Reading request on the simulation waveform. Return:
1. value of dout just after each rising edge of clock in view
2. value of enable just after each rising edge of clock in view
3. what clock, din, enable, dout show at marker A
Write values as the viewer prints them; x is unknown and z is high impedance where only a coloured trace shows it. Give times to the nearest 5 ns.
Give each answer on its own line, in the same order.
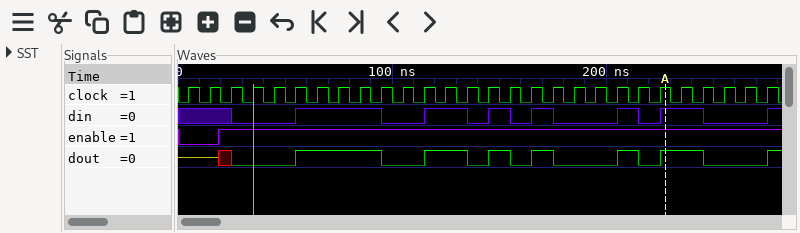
z z 0 0 0 1 1 1 1 0 0 1 1 0 1 0 1 0 0 0 1 0 1 1 0 0 0 1
0 0 1 1 1 1 1 1 1 1 1 1 1 1 1 1 1 1 1 1 1 1 1 1 1 1 1 1
clock=1, din=1, enable=1, dout=1
